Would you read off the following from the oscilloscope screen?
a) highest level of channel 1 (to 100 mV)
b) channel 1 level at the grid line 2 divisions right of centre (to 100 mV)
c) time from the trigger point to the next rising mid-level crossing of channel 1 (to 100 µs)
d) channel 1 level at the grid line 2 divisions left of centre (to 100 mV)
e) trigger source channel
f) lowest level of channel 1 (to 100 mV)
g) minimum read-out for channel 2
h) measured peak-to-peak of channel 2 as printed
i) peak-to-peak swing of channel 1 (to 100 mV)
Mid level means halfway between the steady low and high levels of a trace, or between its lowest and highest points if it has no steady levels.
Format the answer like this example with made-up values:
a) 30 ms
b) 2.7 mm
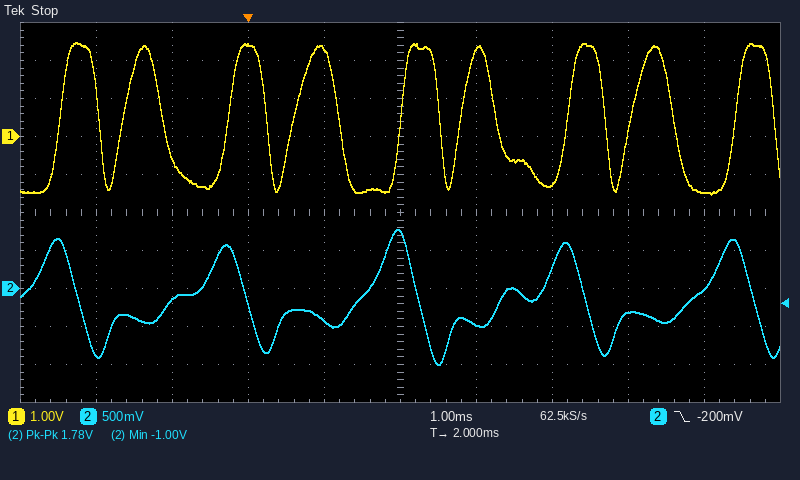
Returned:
a) 2.5 V
b) -1.2 V
c) 600 µs
d) 2.4 V
e) channel 2
f) -1.5 V
g) -1.00 V
h) 1.78 V
i) 4.0 V
